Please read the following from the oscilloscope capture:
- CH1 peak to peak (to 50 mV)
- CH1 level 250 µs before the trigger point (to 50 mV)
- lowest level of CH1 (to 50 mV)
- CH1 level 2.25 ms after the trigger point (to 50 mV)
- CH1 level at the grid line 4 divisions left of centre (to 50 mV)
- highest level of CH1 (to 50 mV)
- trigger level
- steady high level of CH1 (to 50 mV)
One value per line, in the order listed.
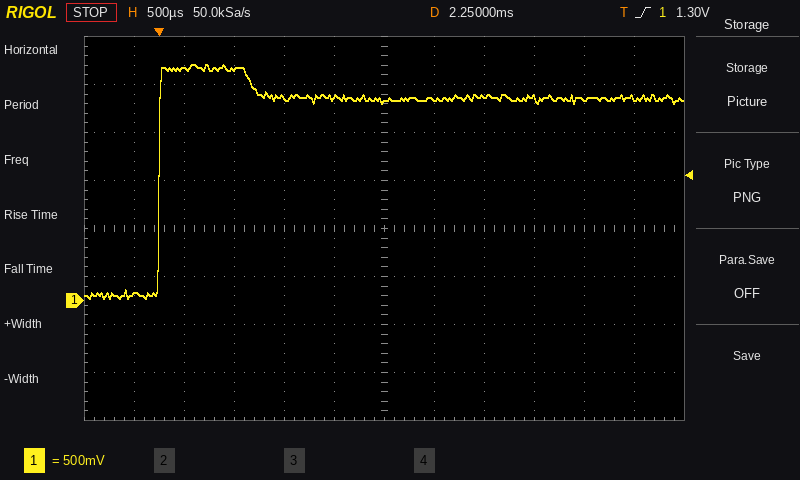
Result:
2.45 V
50 mV
0 mV
2.05 V
2.40 V
2.45 V
1.30 V
2.10 V
